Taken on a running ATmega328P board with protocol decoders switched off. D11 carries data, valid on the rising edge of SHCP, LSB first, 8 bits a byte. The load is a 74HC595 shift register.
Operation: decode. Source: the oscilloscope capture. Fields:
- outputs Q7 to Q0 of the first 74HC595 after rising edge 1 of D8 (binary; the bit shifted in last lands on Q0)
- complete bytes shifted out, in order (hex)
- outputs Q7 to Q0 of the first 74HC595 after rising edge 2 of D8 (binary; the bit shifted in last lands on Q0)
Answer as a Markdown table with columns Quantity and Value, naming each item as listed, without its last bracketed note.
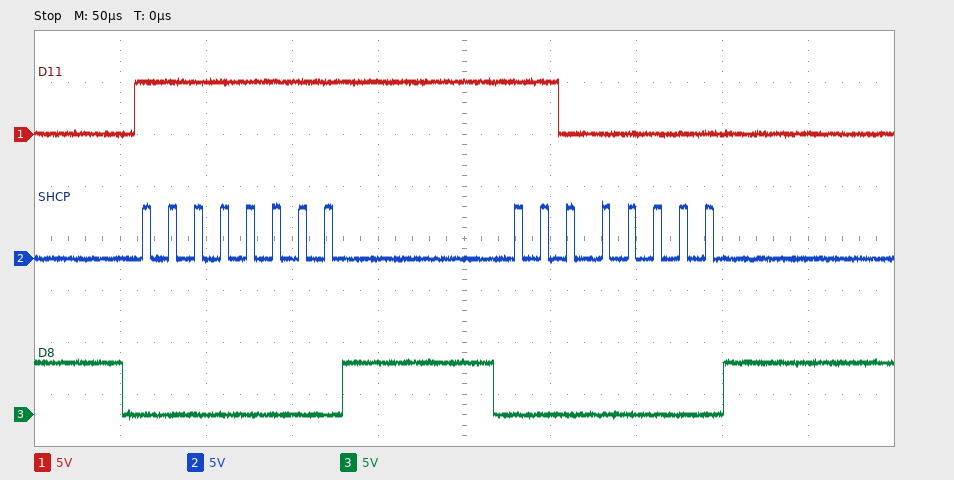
| Quantity | Value |
|---|---|
| outputs Q7 to Q0 of the first 74HC595 after rising edge 1 of D8 | 11111111 |
| complete bytes shifted out, in order | FF 03 |
| outputs Q7 to Q0 of the first 74HC595 after rising edge 2 of D8 | 11000000 |
